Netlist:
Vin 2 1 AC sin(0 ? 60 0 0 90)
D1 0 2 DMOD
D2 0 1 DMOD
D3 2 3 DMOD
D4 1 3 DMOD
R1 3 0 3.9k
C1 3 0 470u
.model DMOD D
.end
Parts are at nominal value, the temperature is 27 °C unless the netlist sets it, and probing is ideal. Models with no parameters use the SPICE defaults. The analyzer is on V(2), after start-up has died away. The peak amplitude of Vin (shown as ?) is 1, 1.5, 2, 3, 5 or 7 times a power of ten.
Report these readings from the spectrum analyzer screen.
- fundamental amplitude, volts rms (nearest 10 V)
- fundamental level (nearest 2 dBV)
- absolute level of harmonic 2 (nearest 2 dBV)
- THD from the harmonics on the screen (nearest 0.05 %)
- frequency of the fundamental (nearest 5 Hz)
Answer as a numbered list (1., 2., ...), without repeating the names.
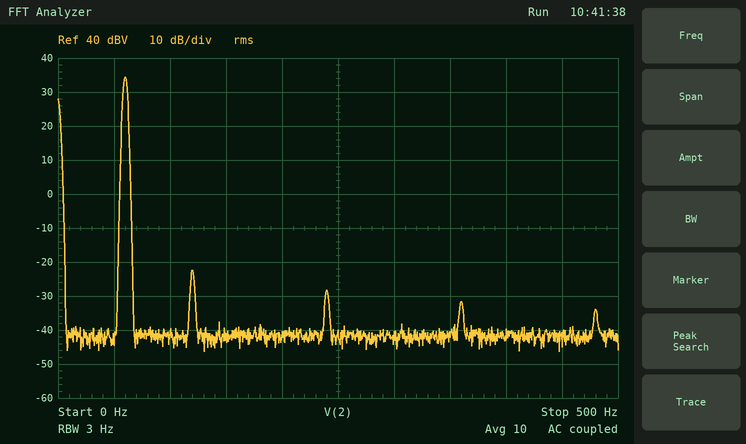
1. 50 V
2. 34 dBV
3. -22 dBV
4. 0.15 %
5. 60 Hz
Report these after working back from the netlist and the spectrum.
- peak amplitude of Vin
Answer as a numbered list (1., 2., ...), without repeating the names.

1. 150 V
